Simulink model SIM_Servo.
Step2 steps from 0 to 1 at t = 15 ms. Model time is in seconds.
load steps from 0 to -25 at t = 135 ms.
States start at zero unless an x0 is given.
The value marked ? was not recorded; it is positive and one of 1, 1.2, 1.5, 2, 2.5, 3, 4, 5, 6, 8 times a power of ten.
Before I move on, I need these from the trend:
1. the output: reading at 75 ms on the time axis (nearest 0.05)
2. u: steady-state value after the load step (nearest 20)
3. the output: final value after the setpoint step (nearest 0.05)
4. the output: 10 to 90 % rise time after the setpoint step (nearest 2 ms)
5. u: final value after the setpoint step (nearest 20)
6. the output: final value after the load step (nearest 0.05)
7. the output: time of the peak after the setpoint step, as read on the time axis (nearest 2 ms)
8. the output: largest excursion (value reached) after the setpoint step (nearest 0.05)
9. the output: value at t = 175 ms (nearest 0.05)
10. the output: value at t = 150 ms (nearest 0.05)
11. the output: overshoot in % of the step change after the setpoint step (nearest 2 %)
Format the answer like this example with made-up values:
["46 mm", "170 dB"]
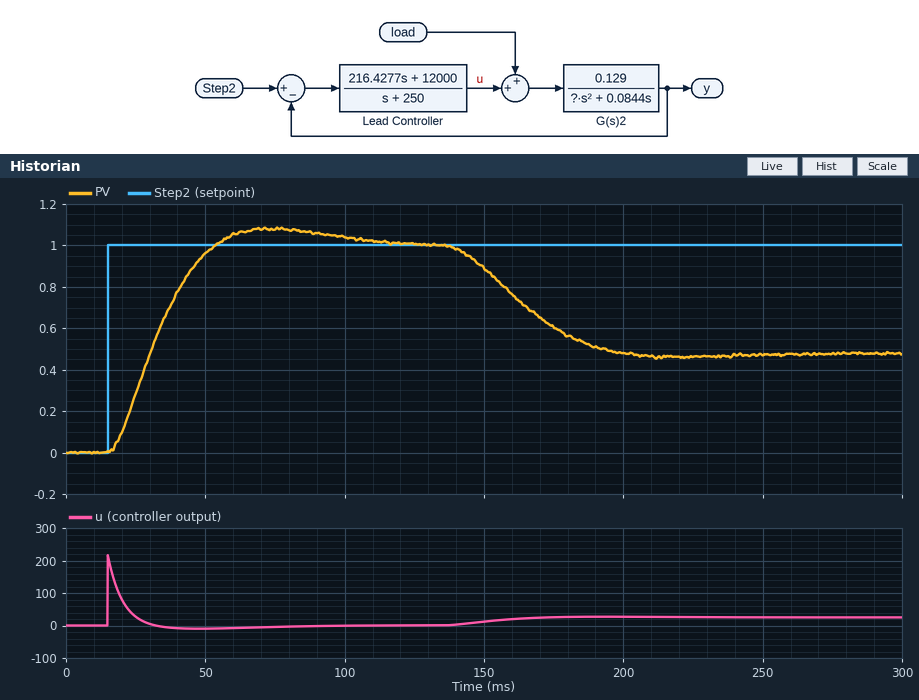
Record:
["1.10", "20", "1.00", "26 ms", "0", "0.50", "74 ms", "1.10", "0.60", "0.90", "8 %"]
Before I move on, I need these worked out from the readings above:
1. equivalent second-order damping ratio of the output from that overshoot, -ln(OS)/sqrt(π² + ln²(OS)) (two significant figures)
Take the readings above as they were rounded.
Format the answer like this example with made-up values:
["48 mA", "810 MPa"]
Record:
["0.63"]
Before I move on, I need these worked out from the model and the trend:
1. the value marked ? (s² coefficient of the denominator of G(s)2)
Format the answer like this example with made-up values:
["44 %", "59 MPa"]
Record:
["0.0025"]
